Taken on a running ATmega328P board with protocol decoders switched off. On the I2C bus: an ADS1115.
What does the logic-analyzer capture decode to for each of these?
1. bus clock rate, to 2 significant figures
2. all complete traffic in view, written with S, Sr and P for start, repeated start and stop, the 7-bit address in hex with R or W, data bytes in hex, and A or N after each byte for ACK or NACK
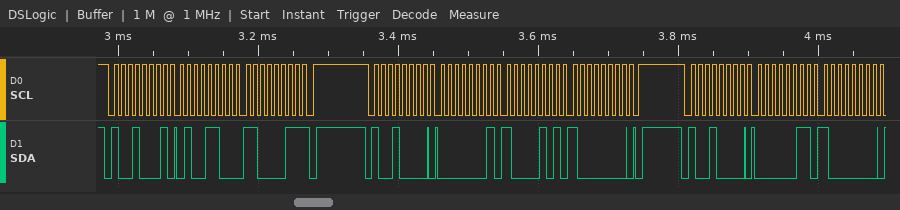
100 kHz
S 48R A 4C A C3 N P S 48W A 01 A 85 A 80 A P S 48W A 03 A 80 A
